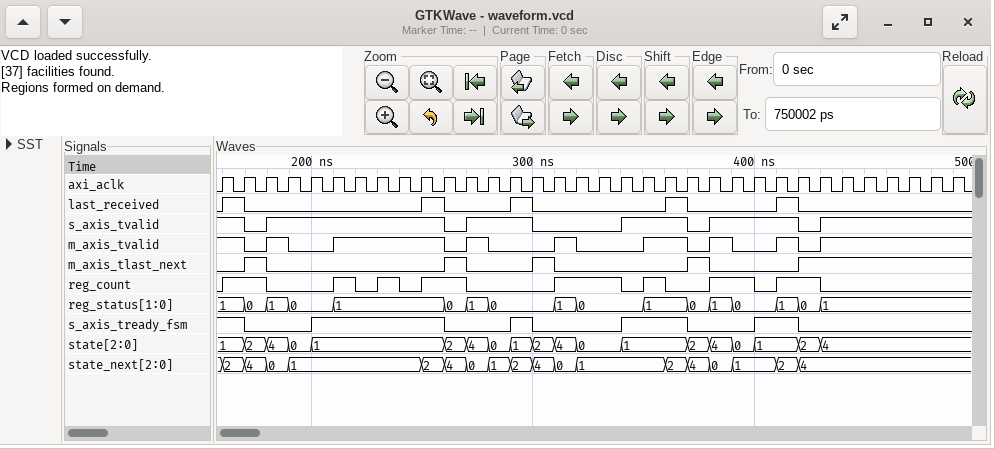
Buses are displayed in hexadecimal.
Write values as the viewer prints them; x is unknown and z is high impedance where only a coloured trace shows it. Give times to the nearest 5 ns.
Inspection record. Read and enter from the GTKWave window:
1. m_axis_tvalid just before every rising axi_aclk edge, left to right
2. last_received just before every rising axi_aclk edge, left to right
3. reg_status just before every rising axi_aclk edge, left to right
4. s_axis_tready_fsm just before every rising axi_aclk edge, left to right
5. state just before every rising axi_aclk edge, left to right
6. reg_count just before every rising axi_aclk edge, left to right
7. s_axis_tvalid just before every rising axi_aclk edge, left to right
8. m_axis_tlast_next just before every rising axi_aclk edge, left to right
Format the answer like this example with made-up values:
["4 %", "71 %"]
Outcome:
["1 1 0 1 0 0 1 1 1 1 1 0 1 0 0 0 1 0 0 0 1 1 0 1 0 0 1 0 1 1 1 1 1 1", "0 1 0 0 0 0 0 0 0 0 1 0 0 0 1 0 0 0 0 0 0 1 0 0 0 0 1 0 0 0 0 0 0 0", "1, 1, 0, 1, 0, 0, 1, 1, 1, 1, 1, 0, 1, 0, 0, 0, 1, 0, 0, 0, 1, 1, 0, 1, 0, 0, 1, 0, 1, 1, 1, 1, 1, 1", "1 1 0 0 0 1 1 1 1 1 1 0 0 0 1 0 0 0 0 1 1 1 0 0 0 1 1 0 0 0 0 0 0 0", "1, 1, 2, 4, 0, 1, 1, 1, 1, 1, 1, 2, 4, 0, 1, 2, 4, 0, 0, 1, 1, 1, 2, 4, 0, 1, 1, 2, 4, 4, 4, 4, 4, 4", "0 1 1 0 0 0 1 0 1 0 1 1 0 0 0 0 1 1 1 0 1 0 0 1 1 0 1 1 0 0 0 0 0 0", "1 1 0 1 1 1 1 1 1 1 1 0 1 1 1 0 0 0 0 1 1 1 0 1 1 1 1 0 1 1 1 1 1 1", "0 0 1 0 0 0 0 0 0 0 0 1 0 0 0 1 0 0 0 0 0 0 1 0 0 0 0 1 1 1 1 1 1 1"]
